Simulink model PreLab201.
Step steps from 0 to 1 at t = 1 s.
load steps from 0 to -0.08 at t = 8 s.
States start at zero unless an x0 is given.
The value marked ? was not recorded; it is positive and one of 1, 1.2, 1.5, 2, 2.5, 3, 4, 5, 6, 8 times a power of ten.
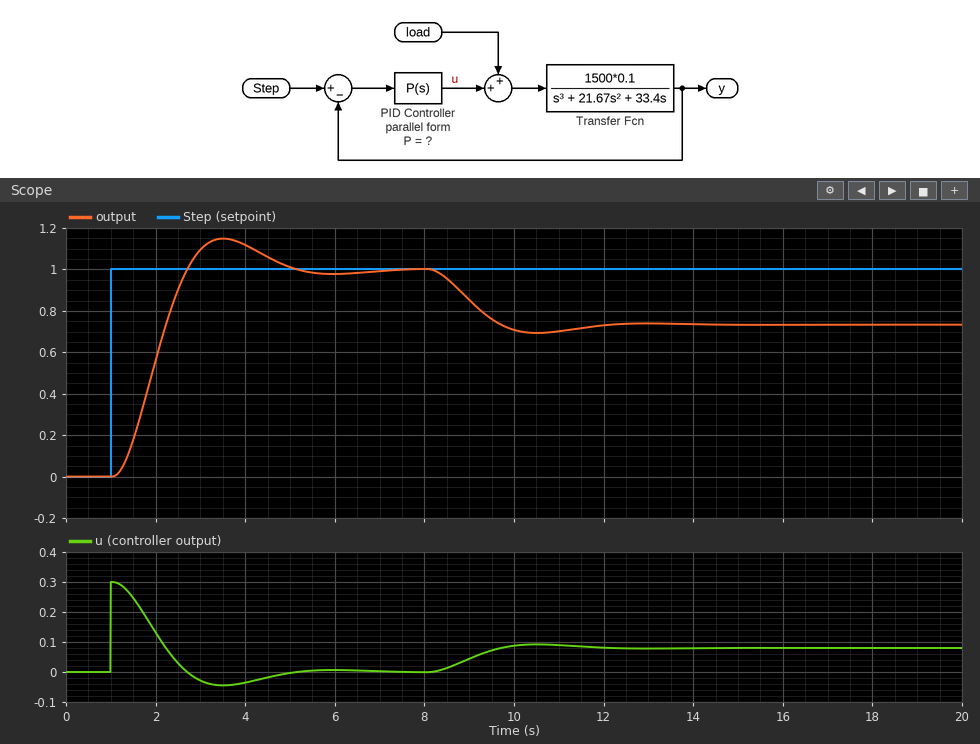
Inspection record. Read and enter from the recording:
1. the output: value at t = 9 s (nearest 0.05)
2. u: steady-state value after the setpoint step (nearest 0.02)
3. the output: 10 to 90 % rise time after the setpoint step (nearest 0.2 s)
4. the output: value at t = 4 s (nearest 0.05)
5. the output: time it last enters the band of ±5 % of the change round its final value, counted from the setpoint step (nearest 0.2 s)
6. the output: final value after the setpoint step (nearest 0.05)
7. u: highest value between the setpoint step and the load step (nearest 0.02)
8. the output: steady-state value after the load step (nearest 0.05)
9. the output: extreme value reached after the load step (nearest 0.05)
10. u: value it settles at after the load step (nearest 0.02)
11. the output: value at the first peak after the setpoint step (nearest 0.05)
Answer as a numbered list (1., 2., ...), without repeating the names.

1. 0.85
2. 0.00
3. 1.2 s
4. 1.10
5. 3.6 s
6. 1.00
7. 0.30
8. 0.75
9. 0.70
10. 0.08
11. 1.15
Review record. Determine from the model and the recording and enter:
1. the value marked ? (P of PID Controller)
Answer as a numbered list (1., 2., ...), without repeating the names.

1. 0.3
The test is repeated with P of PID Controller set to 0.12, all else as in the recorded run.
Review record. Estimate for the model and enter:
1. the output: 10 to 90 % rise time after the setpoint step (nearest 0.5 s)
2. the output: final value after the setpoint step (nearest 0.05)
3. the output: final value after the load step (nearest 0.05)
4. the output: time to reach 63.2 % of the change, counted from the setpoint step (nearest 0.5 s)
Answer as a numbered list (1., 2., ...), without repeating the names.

1. 3.0 s
2. 1.00
3. 0.35
4. 2.0 s
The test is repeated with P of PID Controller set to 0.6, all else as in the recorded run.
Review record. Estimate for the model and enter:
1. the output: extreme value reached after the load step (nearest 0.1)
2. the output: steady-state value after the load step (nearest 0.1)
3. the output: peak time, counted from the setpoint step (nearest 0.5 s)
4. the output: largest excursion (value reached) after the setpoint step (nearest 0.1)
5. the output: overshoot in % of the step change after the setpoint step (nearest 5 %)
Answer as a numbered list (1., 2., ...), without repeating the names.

1. 0.8
2. 0.9
3. 1.5 s
4. 1.3
5. 30 %
